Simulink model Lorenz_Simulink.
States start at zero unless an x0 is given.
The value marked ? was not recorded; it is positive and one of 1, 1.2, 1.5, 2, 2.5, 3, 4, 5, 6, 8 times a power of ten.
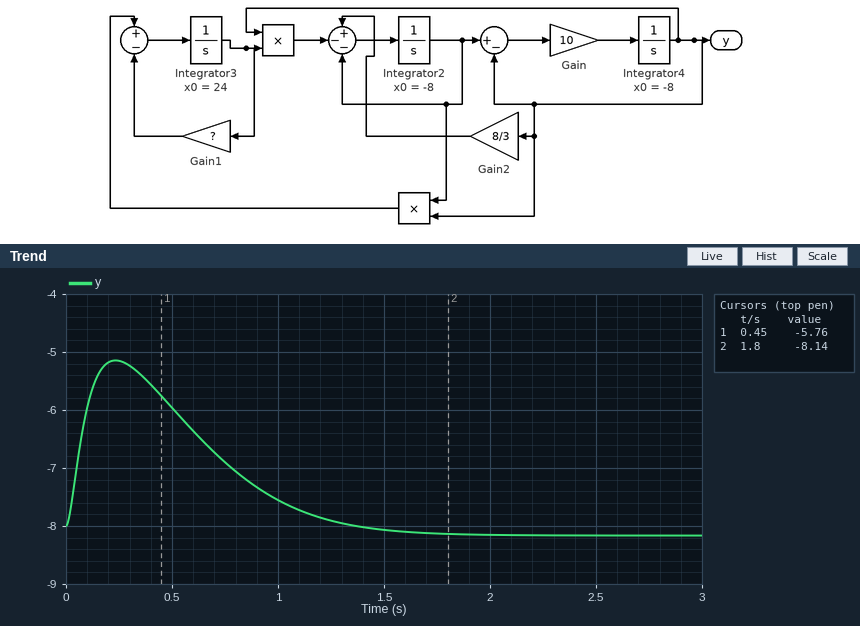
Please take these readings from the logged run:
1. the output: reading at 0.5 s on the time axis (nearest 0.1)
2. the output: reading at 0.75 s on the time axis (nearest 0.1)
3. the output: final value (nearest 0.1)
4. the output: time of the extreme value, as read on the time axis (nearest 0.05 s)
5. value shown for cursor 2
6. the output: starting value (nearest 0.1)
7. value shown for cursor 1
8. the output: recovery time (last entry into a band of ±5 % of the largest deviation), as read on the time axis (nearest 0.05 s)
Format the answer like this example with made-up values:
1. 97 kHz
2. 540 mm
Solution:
1. -6.0
2. -6.9
3. -8.2
4. 0.25 s
5. -8.14
6. -8.0
7. -5.76
8. 1.40 s
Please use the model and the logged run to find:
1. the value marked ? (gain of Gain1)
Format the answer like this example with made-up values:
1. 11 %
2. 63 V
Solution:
1. 40
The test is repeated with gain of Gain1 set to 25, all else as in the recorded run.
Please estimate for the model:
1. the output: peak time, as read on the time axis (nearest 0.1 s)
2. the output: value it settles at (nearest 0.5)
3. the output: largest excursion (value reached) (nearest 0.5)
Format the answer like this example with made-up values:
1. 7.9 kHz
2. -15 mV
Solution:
1. 0.3 s
2. -6.5
3. -3.0
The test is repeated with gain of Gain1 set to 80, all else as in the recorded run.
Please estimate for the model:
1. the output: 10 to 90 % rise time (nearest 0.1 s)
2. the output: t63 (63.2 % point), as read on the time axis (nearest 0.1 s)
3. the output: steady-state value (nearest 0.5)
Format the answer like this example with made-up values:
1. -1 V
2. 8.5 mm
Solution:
1. 0.8 s
2. 0.8 s
3. -11.5
